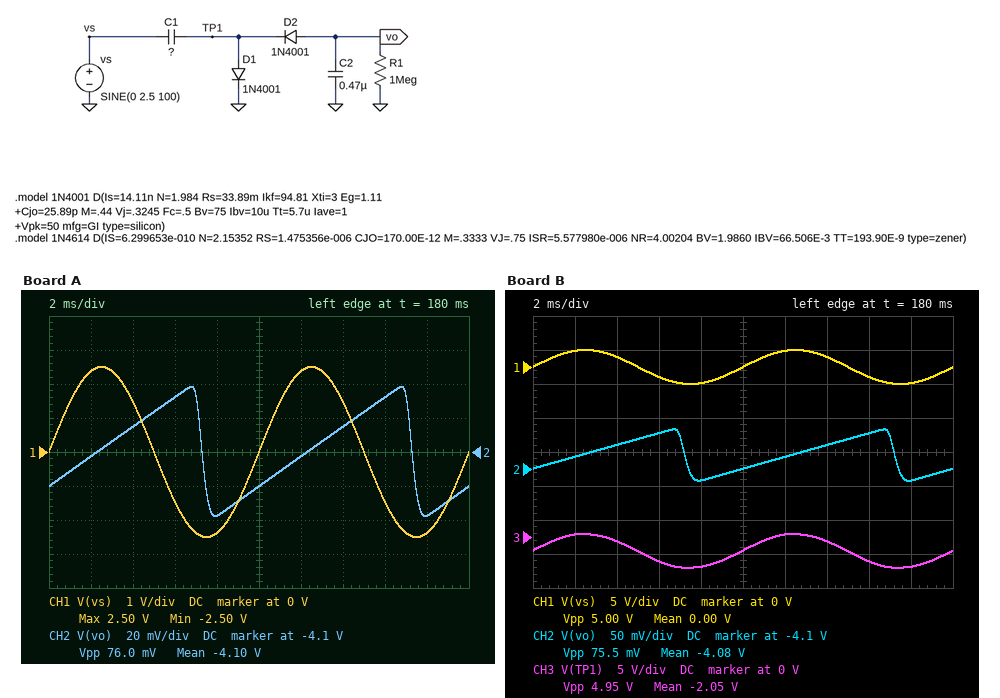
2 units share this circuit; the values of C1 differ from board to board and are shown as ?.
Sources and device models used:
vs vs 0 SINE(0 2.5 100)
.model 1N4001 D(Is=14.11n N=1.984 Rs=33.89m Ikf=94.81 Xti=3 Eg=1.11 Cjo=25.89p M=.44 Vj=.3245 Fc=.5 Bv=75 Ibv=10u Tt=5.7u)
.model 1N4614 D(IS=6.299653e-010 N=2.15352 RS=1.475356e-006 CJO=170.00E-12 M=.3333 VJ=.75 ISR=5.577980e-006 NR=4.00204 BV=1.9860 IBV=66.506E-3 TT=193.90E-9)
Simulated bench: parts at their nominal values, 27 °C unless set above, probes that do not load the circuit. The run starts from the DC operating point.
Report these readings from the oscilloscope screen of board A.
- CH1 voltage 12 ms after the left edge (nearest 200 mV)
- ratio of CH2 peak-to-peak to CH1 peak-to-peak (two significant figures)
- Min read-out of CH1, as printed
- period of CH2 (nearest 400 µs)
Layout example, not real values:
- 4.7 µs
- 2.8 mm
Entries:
- 2.4 V
- 0.015
- -2.50 V
- 10.0 ms
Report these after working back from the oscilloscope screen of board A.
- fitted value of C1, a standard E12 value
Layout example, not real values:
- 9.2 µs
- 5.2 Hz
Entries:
- 560 nF
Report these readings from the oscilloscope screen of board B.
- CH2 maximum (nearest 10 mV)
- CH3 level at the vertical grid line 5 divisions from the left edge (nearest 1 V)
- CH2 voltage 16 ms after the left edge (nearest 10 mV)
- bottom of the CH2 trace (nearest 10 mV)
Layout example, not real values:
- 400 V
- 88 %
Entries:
- -4.04 V
- -2 V
- -4.05 V
- -4.12 V
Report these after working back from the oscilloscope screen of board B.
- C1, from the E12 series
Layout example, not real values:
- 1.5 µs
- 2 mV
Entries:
- 330 nF
